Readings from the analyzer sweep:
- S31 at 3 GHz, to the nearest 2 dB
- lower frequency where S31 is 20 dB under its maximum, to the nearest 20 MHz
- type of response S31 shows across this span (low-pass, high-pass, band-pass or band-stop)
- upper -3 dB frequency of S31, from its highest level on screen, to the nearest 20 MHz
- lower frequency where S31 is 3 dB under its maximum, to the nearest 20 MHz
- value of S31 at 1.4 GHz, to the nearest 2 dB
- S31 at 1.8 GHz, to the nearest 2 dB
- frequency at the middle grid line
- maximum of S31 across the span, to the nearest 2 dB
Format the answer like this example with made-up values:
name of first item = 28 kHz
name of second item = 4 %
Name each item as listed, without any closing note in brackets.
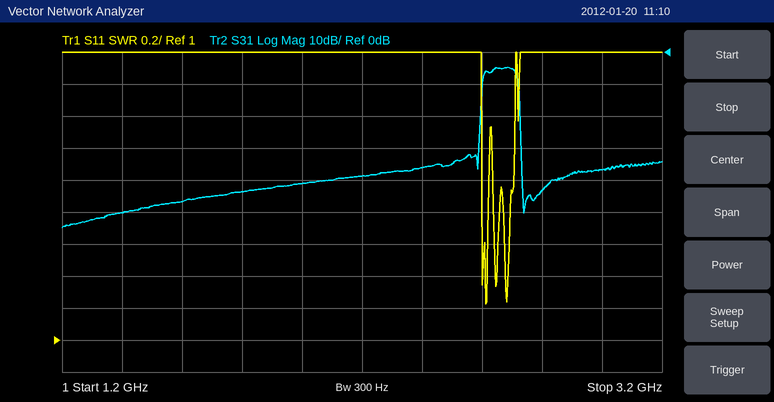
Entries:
S31 at 3 GHz, to the nearest 2 dB = -36 dB
lower frequency where S31 is 20 dB under its maximum, to the nearest 20 MHz = 2.60 GHz
type of response S31 shows across this span = band-pass
upper -3 dB frequency of S31, from its highest level on screen, to the nearest 20 MHz = 2.72 GHz
lower frequency where S31 is 3 dB under its maximum, to the nearest 20 MHz = 2.60 GHz
value of S31 at 1.4 GHz, to the nearest 2 dB = -50 dB
S31 at 1.8 GHz, to the nearest 2 dB = -44 dB
frequency at the middle grid line = 2.2 GHz
maximum of S31 across the span, to the nearest 2 dB = -4 dB
